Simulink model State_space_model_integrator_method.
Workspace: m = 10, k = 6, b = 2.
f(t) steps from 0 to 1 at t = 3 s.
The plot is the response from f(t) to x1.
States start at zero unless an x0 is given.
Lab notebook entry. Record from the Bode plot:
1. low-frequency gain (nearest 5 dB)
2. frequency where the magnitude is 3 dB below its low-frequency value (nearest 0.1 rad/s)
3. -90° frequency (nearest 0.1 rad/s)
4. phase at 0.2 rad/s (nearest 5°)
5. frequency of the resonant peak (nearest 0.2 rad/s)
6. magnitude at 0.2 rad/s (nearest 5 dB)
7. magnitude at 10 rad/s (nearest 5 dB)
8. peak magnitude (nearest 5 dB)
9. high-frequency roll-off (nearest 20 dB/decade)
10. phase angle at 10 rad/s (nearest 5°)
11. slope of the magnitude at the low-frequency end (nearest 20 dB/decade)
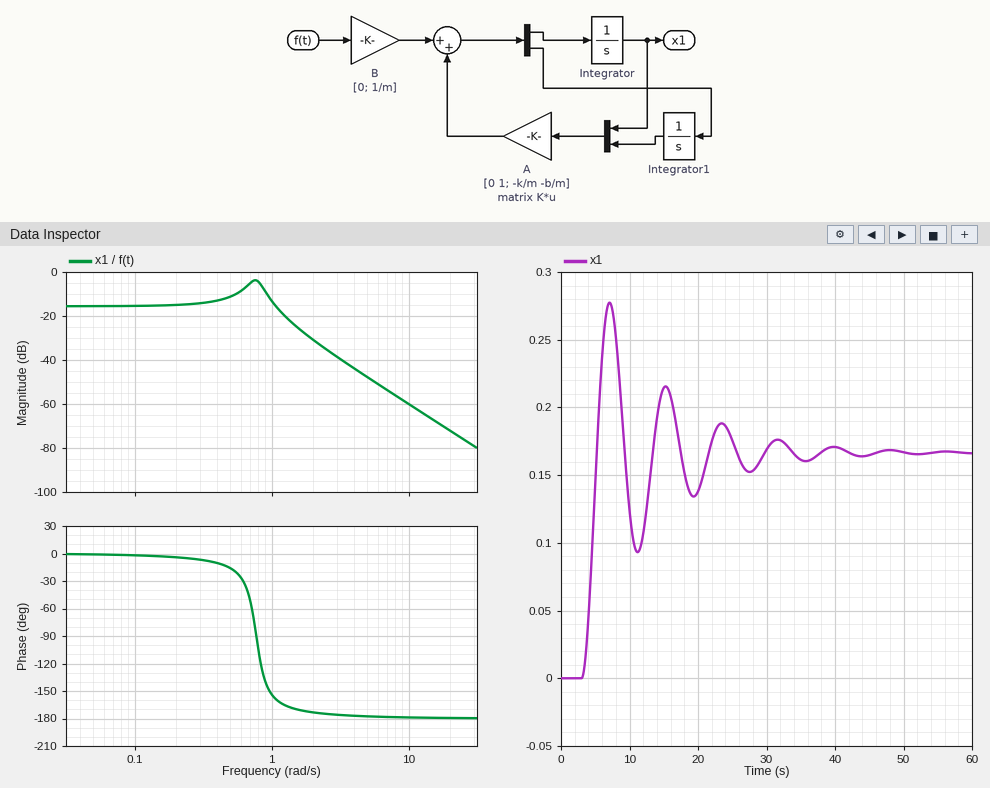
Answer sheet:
-15 dB
1.2 rad/s
0.8 rad/s
-5°
0.8 rad/s
-15 dB
-60 dB
-5 dB
-40 dB/decade
-180°
0 dB/decade
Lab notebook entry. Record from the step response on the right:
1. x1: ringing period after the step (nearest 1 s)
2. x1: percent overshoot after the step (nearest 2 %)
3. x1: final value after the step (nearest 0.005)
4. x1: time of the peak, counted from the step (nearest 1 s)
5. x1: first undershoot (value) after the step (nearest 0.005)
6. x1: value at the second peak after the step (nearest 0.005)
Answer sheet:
8 s
66 %
0.165
4 s
0.095
0.215
